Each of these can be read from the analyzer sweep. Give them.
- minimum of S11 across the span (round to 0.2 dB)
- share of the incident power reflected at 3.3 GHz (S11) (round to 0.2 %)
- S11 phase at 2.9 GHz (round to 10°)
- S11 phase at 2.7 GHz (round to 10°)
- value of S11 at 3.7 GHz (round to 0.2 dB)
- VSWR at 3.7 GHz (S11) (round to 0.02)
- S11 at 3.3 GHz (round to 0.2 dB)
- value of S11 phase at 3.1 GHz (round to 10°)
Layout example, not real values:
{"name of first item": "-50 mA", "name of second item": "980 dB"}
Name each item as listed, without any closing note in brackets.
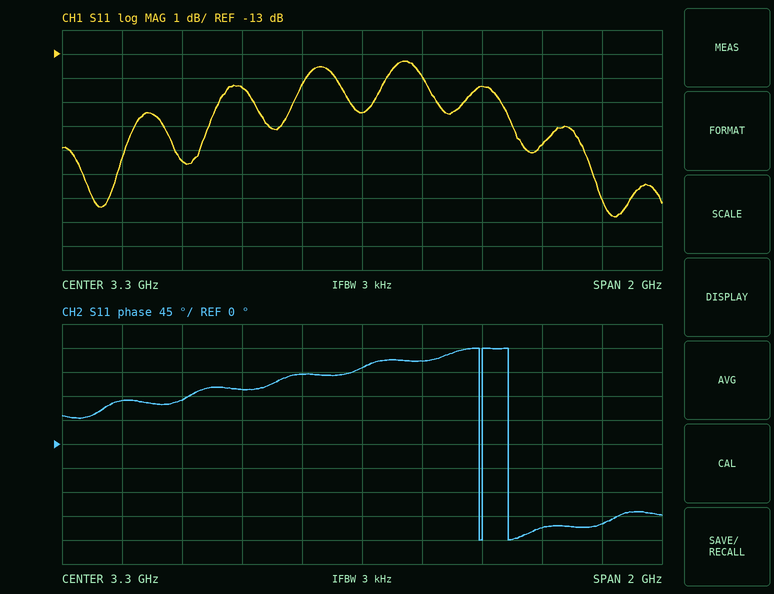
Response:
{"minimum of S11 across the span": "-19.8 dB", "share of the incident power reflected at 3.3 GHz (S11)": "2.8 %", "S11 phase at 2.9 GHz": "100°", "S11 phase at 2.7 GHz": "80°", "value of S11 at 3.7 GHz": "-14.4 dB", "VSWR at 3.7 GHz (S11)": "1.48", "S11 at 3.3 GHz": "-15.4 dB", "value of S11 phase at 3.1 GHz": "130°"}
